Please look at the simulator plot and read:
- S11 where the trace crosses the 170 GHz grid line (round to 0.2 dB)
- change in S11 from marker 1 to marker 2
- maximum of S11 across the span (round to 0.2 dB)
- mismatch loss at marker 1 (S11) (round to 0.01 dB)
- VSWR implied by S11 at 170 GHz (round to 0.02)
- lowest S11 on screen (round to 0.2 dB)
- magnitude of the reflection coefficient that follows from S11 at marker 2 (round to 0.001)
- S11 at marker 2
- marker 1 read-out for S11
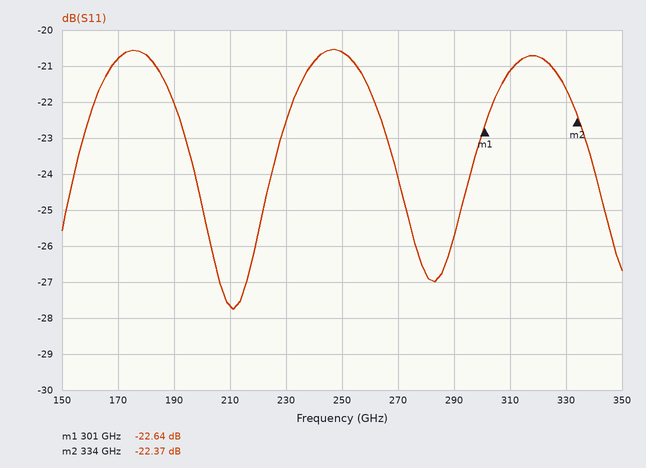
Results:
-20.8 dB
0.27 dB
-20.6 dB
0.02 dB
1.20
-27.8 dB
0.076
-22.37 dB
-22.64 dB
